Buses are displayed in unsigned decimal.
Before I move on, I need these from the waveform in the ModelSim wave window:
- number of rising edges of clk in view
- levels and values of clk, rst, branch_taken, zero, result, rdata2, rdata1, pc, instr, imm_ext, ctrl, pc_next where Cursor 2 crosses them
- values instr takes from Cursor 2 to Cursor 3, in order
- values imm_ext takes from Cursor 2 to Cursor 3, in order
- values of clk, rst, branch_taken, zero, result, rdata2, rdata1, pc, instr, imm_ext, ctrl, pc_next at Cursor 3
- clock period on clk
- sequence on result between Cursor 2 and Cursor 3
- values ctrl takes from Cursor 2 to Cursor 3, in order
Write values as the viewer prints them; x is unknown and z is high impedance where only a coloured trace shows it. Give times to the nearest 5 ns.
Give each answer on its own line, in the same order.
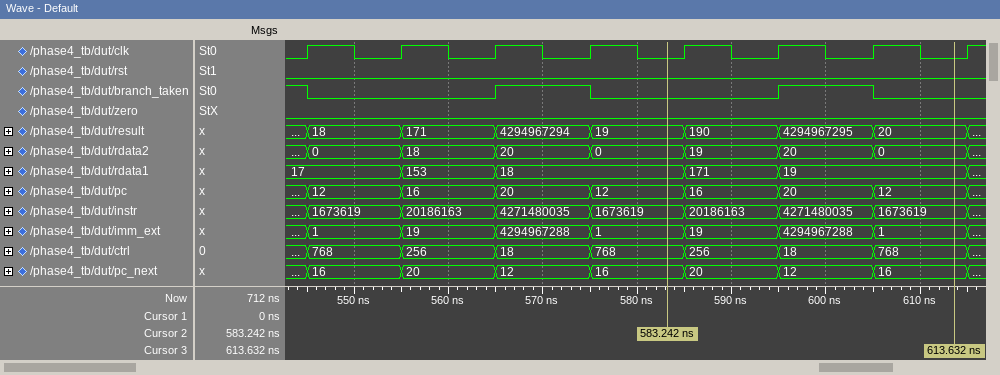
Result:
8
clk=0, rst=0, branch_taken=0, zero=0, result=19, rdata2=0, rdata1=18, pc=12, instr=1673619, imm_ext=1, ctrl=768, pc_next=16
1673619, 20186163, 4271480035, 1673619
1, 19, 4294967288, 1
clk=0, rst=0, branch_taken=0, zero=0, result=20, rdata2=0, rdata1=19, pc=12, instr=1673619, imm_ext=1, ctrl=768, pc_next=16
10 ns
19, 190, 4294967295, 20
768, 256, 18, 768
